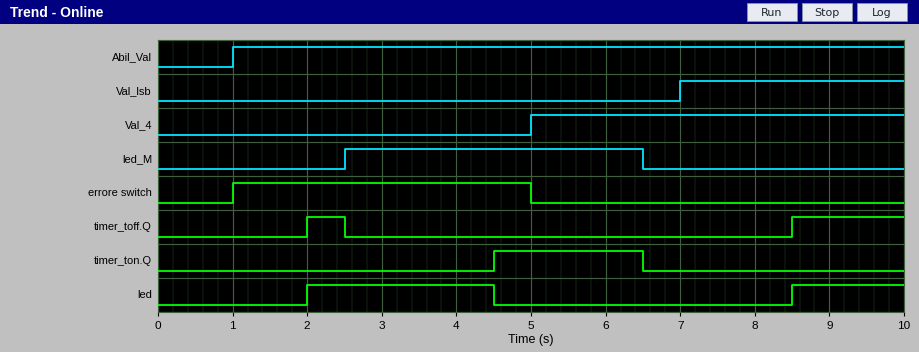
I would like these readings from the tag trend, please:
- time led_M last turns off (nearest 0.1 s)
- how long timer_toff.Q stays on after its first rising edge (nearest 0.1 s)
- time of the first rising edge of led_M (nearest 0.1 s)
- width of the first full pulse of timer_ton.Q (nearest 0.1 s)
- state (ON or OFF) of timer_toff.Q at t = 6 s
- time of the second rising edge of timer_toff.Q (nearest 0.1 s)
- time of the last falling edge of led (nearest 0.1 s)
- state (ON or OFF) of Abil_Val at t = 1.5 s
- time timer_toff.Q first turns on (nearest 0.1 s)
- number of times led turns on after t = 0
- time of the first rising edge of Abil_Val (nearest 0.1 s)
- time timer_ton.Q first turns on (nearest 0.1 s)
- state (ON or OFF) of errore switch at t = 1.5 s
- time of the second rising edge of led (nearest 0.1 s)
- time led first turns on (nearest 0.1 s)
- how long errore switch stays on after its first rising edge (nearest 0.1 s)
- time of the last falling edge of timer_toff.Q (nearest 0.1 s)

6.5 s
0.5 s
2.5 s
2.0 s
OFF
8.5 s
4.5 s
ON
2.0 s
2
1.0 s
4.5 s
ON
8.5 s
2.0 s
4.0 s
2.5 s
